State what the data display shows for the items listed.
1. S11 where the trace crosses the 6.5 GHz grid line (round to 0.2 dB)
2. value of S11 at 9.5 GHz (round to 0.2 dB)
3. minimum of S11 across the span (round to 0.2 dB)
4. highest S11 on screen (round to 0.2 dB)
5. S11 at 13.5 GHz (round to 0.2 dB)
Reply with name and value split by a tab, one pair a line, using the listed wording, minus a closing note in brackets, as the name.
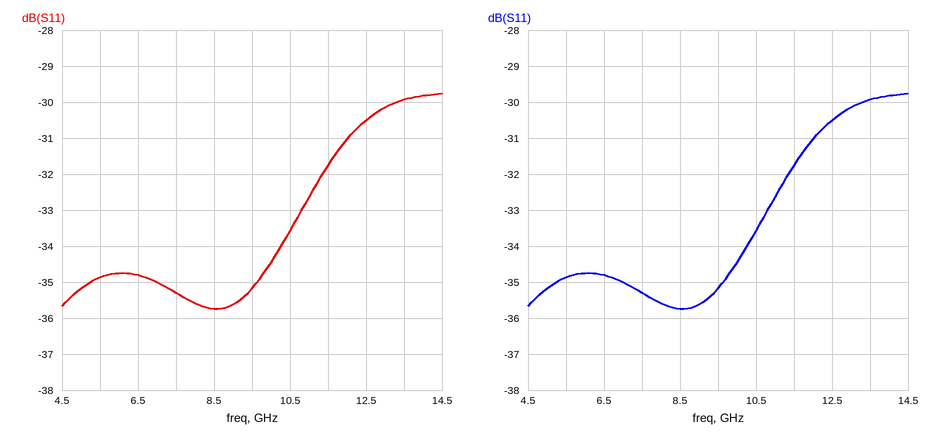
S11 where the trace crosses the 6.5 GHz grid line	-34.8 dB
value of S11 at 9.5 GHz	-35.2 dB
minimum of S11 across the span	-35.8 dB
highest S11 on screen	-29.8 dB
S11 at 13.5 GHz	-30.0 dB
